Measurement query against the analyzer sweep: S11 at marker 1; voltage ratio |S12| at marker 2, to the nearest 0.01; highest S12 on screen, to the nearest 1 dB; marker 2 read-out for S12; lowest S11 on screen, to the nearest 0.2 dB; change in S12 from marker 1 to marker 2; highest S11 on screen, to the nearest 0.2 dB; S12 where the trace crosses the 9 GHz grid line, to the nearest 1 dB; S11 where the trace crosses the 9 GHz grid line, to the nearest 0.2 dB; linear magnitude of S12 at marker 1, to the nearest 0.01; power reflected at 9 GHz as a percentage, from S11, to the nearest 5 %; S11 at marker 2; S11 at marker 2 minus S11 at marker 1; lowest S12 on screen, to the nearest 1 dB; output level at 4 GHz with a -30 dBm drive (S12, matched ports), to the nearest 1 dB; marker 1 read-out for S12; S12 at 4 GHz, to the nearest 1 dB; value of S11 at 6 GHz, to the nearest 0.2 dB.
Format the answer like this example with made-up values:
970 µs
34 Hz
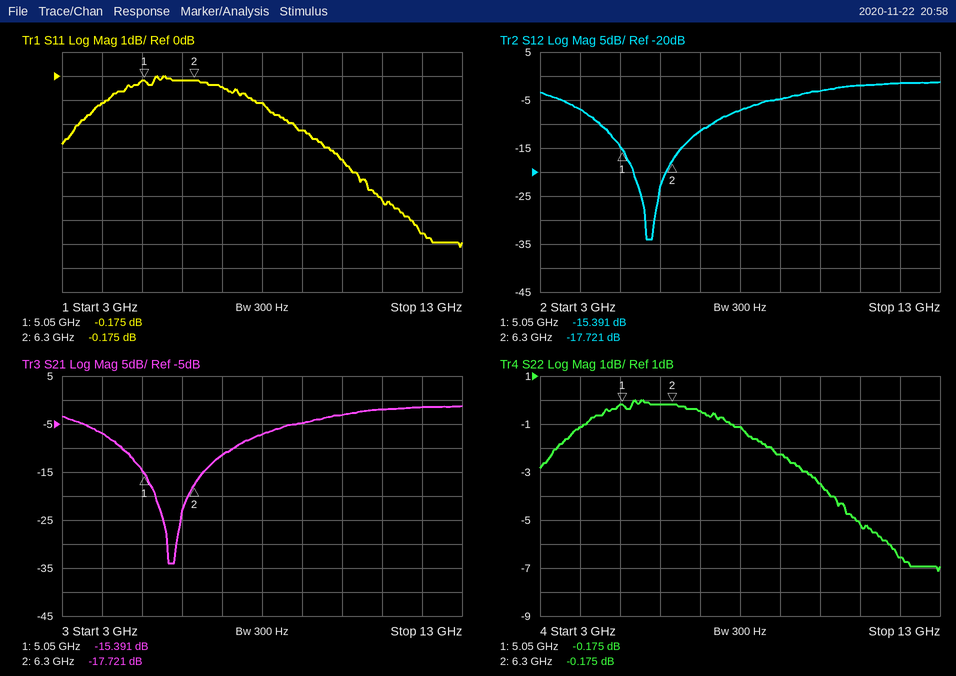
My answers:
-0.175 dB
0.13
-1 dB
-17.721 dB
-7.2 dB
-2.330 dB
0.0 dB
-5 dB
-2.2 dB
0.17
60 %
-0.175 dB
0.000 dB
-34 dB
-37 dBm
-15.391 dB
-7 dB
-0.2 dB
